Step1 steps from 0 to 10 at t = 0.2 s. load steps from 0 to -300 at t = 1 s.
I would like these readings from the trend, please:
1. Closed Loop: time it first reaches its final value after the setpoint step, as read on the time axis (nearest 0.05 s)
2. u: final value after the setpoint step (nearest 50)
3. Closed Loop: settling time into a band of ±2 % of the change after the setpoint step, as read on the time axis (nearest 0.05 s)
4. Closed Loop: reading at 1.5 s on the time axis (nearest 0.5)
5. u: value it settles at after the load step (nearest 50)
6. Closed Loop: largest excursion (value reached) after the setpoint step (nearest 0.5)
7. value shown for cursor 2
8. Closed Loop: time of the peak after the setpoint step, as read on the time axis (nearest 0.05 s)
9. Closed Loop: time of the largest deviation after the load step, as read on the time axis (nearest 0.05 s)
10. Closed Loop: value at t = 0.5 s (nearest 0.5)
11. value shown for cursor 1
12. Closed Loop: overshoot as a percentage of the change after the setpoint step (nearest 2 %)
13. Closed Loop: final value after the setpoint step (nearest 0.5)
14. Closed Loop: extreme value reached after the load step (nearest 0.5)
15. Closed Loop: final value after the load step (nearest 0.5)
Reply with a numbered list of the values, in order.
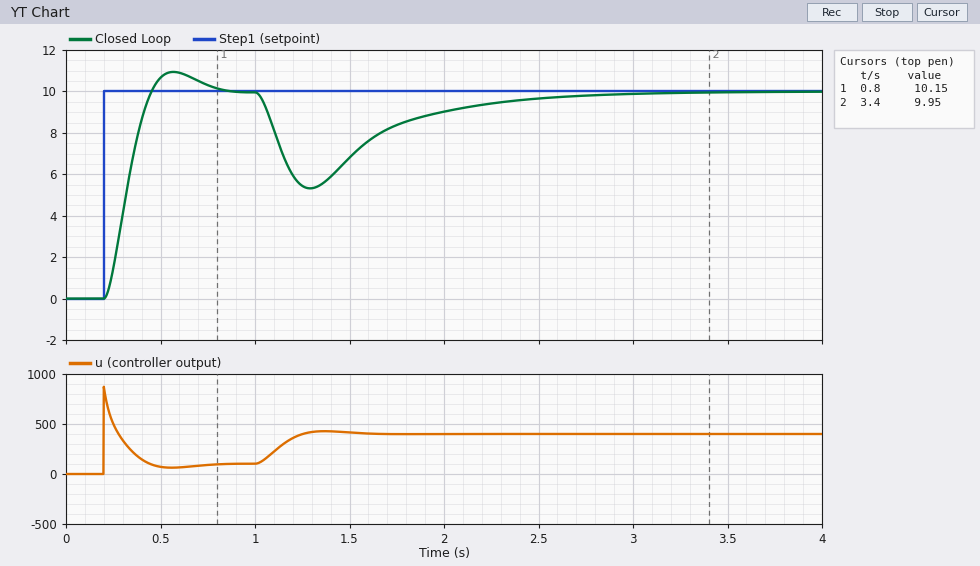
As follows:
1. 0.45 s
2. 100
3. 0.80 s
4. 7.0
5. 400
6. 11.0
7. 9.95
8. 0.55 s
9. 1.30 s
10. 10.5
11. 10.15
12. 10 %
13. 10.0
14. 5.5
15. 10.0
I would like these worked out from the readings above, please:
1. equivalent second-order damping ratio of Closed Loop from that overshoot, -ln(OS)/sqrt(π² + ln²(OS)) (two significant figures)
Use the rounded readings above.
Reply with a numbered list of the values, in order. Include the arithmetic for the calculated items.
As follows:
1. ln(0.1) = -2.303; 2.303 / sqrt(9.870 + 5.302) = 0.59
